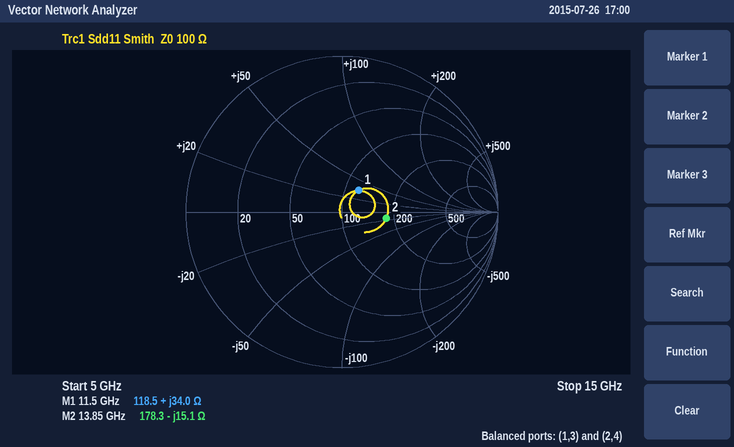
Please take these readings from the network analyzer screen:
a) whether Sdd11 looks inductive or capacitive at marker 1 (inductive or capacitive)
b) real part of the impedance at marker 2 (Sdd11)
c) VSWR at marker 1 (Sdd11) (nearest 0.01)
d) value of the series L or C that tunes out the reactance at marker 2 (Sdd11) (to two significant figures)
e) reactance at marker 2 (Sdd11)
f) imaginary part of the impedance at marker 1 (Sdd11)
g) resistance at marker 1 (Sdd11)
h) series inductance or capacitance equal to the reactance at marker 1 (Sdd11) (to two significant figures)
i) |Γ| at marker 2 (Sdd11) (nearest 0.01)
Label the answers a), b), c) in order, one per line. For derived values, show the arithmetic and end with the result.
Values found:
a) inductive
b) 178.3 Ω
c) 1.42
d) L = 15.1 Ω/(2π × 13.85 GHz) ≈ 174 pH, so 170 pH to two significant figures
e) -15.1 Ω
f) +34.0 Ω
g) 118.5 Ω
h) L = 34 Ω/(2π × 11.5 GHz) ≈ 471 pH, so 470 pH to two significant figures
i) 0.29
